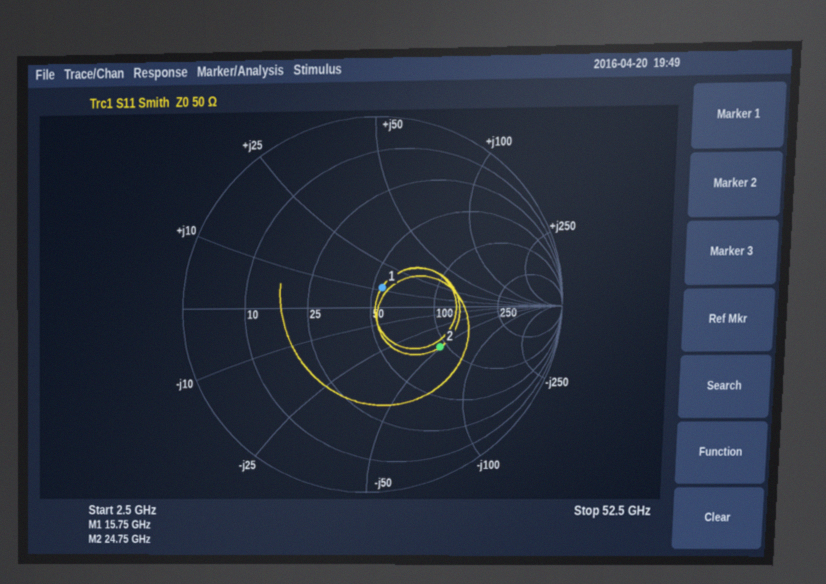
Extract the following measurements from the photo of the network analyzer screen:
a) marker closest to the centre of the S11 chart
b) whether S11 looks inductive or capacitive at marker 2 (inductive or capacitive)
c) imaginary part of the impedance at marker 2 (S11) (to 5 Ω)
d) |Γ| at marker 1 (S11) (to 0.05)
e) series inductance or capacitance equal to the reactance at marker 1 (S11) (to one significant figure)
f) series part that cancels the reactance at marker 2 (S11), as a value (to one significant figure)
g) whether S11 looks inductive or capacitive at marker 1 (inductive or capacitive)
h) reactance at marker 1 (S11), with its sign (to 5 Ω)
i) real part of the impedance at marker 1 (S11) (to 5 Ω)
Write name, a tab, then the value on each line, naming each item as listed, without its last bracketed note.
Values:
marker closest to the centre of the S11 chart	marker 1
whether S11 looks inductive or capacitive at marker 2	capacitive
imaginary part of the impedance at marker 2 (S11)	-50 Ω
|Γ| at marker 1 (S11)	0.10
series inductance or capacitance equal to the reactance at marker 1 (S11)	100 pH
series part that cancels the reactance at marker 2 (S11), as a value	300 pH
whether S11 looks inductive or capacitive at marker 1	inductive
reactance at marker 1 (S11), with its sign	+10 Ω
real part of the impedance at marker 1 (S11)	55 Ω
